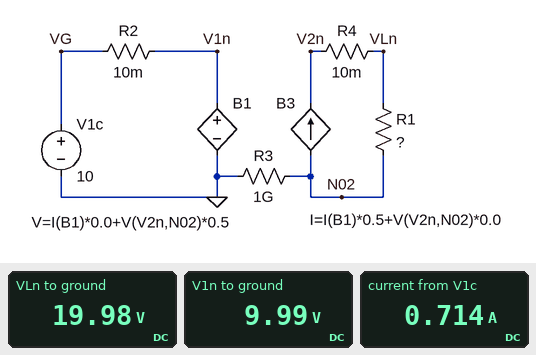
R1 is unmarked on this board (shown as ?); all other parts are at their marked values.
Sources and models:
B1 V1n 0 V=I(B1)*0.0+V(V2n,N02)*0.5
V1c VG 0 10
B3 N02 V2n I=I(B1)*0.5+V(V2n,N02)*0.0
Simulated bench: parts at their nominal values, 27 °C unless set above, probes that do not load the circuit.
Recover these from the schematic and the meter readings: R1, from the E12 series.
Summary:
56 Ω
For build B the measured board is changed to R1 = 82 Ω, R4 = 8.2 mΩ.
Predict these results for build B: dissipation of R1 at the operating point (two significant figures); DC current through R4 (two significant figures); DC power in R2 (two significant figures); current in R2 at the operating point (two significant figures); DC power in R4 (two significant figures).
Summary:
4.9 W
240 mA
2.4 mW
490 mA
490 µW
